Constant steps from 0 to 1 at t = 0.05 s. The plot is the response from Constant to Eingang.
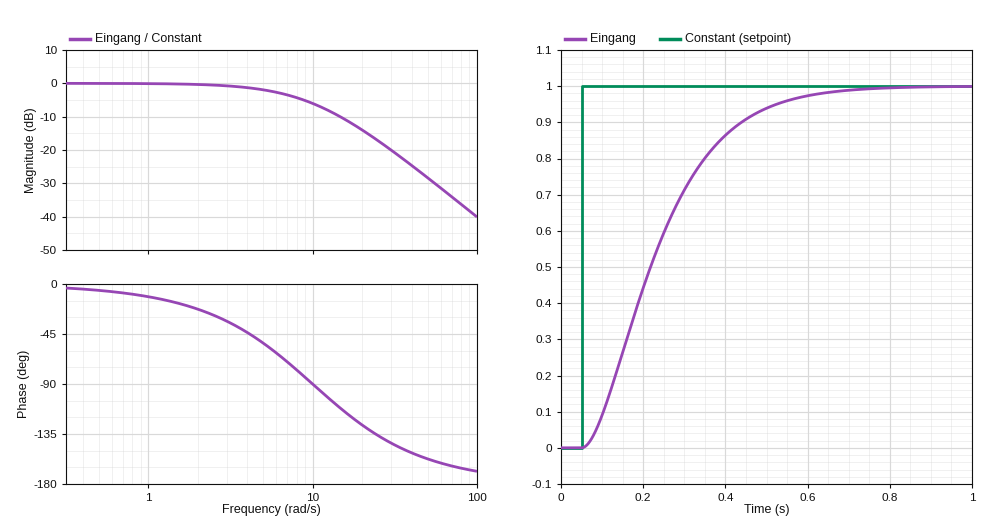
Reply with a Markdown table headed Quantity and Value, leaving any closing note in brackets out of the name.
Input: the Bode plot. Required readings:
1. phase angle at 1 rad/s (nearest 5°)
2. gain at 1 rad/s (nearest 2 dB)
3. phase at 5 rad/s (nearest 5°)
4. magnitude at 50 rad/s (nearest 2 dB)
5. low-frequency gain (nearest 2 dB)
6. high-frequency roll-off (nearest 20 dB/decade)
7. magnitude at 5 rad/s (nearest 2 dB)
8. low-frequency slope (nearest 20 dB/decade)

| Quantity | Value |
|---|---|
| phase angle at 1 rad/s | -10° |
| gain at 1 rad/s | 0 dB |
| phase at 5 rad/s | -55° |
| magnitude at 50 rad/s | -28 dB |
| low-frequency gain | 0 dB |
| high-frequency roll-off | -40 dB/decade |
| magnitude at 5 rad/s | -2 dB |
| low-frequency slope | 0 dB/decade |
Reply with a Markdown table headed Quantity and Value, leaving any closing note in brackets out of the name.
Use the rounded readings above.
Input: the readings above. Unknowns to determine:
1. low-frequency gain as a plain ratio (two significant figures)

| Quantity | Value |
|---|---|
| low-frequency gain as a plain ratio | 1.0 |
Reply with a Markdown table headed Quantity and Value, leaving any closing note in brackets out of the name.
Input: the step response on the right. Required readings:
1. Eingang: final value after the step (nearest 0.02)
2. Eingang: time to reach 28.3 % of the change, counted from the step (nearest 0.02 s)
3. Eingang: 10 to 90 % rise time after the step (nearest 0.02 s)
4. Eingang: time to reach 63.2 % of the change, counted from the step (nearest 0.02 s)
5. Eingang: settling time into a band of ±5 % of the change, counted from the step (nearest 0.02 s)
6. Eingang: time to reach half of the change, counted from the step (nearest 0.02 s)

| Quantity | Value |
|---|---|
| Eingang: final value after the step | 1.00 |
| Eingang: time to reach 28.3 % of the change, counted from the step | 0.10 s |
| Eingang: 10 to 90 % rise time after the step | 0.34 s |
| Eingang: time to reach 63.2 % of the change, counted from the step | 0.22 s |
| Eingang: settling time into a band of ±5 % of the change, counted from the step | 0.48 s |
| Eingang: time to reach half of the change, counted from the step | 0.16 s |
